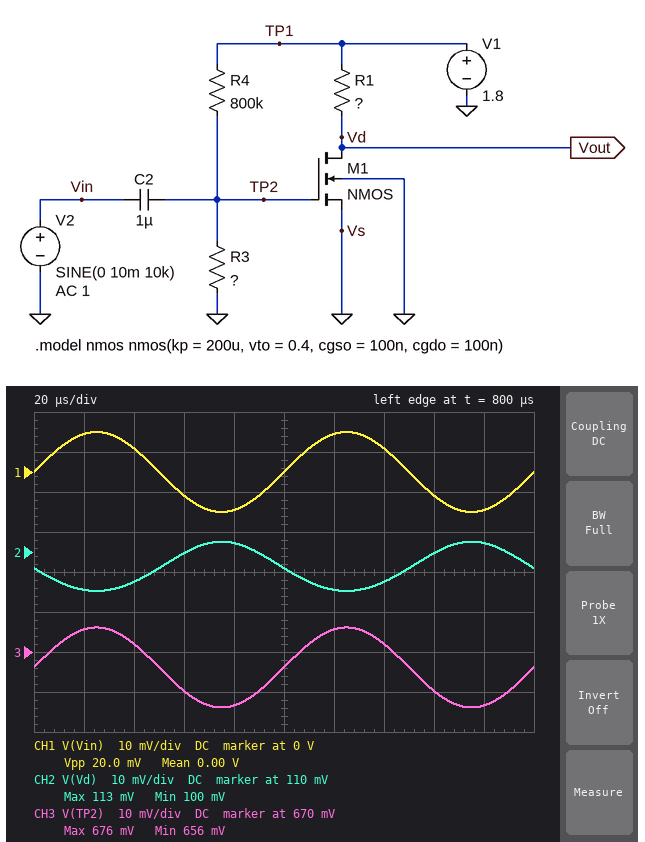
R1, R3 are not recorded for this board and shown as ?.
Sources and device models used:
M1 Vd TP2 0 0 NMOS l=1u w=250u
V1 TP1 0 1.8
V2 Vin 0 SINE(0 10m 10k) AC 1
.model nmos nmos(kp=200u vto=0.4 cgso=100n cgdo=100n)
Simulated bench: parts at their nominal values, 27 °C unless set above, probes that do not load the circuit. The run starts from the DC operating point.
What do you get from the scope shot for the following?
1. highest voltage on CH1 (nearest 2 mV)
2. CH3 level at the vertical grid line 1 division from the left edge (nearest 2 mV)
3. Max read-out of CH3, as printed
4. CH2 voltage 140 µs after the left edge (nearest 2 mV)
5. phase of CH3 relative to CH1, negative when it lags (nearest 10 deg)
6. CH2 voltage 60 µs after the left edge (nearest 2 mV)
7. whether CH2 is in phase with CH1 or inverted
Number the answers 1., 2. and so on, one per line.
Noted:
1. 10 mV
2. 676 mV
3. 676 mV
4. 102 mV
5. 0 deg
6. 110 mV
7. inverted
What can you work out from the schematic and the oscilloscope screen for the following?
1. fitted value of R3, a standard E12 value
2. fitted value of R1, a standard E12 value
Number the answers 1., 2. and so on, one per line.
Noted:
1. 470 kΩ
2. 1.5 kΩ
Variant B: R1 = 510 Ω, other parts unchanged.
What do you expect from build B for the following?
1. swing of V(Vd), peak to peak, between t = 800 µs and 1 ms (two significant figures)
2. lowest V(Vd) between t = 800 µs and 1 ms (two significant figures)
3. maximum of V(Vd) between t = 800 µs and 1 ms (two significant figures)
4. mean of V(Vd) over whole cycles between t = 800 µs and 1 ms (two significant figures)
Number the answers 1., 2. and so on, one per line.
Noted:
1. 140 mV
2. 830 mV
3. 960 mV
4. 900 mV
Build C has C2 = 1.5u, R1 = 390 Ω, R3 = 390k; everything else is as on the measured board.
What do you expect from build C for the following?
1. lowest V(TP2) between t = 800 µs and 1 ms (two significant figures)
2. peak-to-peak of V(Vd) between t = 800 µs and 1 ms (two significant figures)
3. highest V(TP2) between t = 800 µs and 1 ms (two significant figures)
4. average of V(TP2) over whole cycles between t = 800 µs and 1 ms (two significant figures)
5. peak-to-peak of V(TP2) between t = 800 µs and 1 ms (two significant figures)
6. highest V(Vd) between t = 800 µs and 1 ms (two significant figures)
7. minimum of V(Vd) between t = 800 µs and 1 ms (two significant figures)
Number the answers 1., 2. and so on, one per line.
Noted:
1. 580 mV
2. 74 mV
3. 600 mV
4. 590 mV
5. 20 mV
6. 1.5 V
7. 1.4 V
